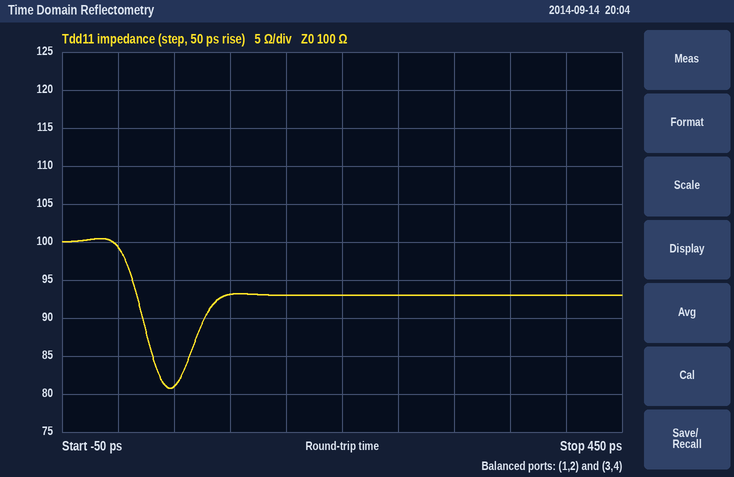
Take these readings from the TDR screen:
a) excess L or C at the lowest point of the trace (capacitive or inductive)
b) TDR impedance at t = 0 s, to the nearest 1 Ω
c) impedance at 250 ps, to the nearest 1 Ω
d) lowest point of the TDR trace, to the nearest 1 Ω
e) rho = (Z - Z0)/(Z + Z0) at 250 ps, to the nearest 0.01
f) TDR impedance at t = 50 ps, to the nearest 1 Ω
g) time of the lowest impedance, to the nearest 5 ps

capacitive
99 Ω
93 Ω
81 Ω
-0.04
81 Ω
45 ps
